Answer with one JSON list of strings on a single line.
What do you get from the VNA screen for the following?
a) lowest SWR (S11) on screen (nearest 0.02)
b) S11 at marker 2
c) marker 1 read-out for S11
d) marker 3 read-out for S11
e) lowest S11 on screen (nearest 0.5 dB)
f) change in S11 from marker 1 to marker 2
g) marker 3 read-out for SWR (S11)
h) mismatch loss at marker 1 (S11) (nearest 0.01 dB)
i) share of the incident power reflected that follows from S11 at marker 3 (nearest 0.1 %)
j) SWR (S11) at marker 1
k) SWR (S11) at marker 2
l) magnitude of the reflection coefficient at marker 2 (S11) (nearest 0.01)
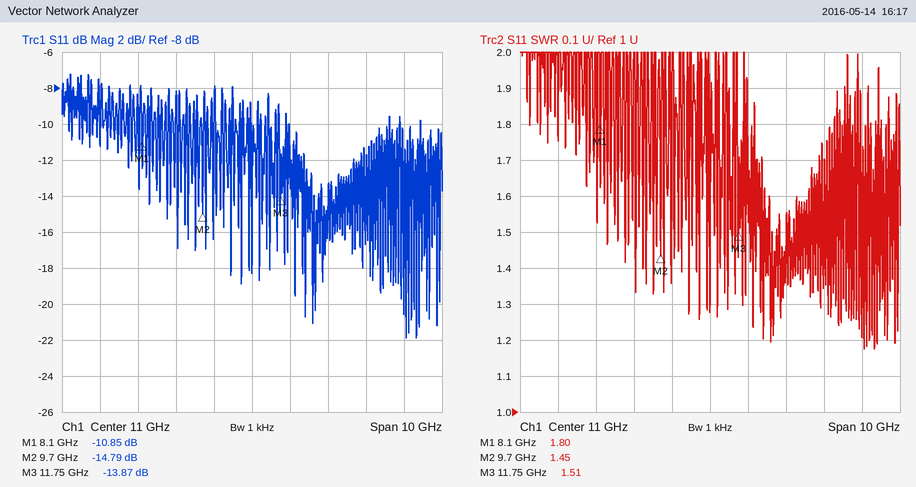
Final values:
["1.18", "-14.79 dB", "-10.85 dB", "-13.87 dB", "-22.0 dB", "-3.94 dB", "1.51", "0.37 dB", "4.1 %", "1.80", "1.45", "0.18"]
